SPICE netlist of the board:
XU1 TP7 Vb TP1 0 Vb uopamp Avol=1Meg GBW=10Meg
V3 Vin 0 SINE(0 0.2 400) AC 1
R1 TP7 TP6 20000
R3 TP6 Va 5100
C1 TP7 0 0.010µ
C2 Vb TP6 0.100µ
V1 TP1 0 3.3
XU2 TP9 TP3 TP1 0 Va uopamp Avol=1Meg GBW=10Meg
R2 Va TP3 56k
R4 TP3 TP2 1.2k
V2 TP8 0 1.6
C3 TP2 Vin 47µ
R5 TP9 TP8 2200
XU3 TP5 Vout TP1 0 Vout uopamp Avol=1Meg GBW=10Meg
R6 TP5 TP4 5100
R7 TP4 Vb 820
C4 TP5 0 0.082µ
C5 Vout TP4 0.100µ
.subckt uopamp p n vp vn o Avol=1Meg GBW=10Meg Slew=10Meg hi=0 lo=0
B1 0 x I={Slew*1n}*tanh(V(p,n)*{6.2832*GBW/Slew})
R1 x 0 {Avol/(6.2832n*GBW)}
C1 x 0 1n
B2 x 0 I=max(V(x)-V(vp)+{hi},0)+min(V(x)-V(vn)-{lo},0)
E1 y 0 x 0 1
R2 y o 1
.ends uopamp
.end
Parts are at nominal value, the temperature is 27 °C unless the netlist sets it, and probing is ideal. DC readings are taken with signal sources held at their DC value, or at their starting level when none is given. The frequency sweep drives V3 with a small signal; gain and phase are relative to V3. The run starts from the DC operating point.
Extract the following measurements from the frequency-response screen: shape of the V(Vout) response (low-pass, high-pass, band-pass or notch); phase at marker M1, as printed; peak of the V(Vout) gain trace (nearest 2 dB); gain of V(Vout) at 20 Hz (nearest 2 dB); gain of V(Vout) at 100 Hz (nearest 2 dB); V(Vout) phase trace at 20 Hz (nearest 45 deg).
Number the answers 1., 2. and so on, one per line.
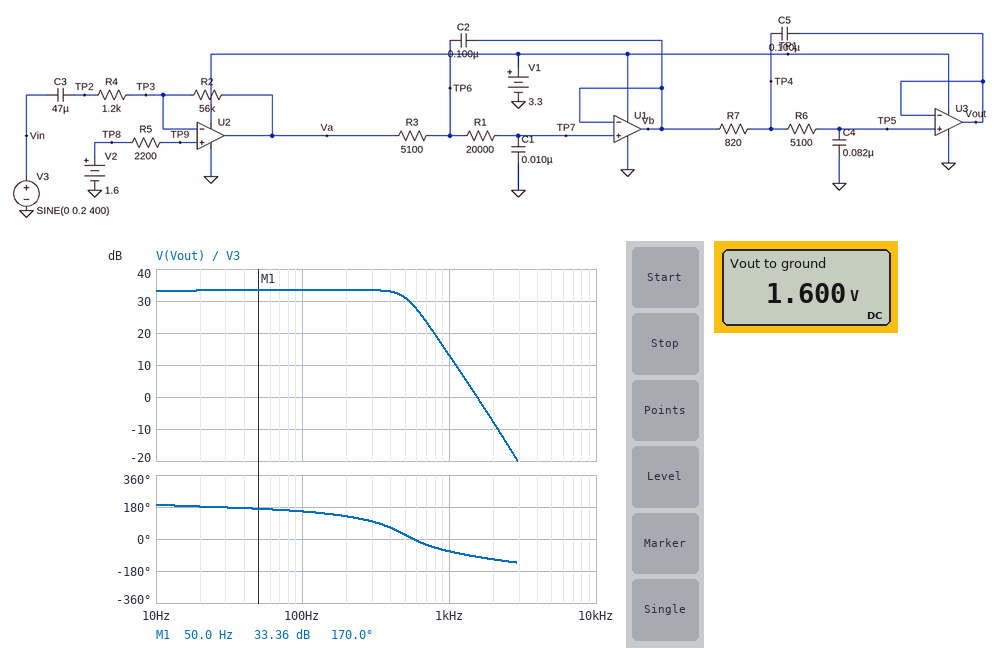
1. low-pass
2. 170.0 deg
3. 34 dB
4. 34 dB
5. 34 dB
6. 180 deg
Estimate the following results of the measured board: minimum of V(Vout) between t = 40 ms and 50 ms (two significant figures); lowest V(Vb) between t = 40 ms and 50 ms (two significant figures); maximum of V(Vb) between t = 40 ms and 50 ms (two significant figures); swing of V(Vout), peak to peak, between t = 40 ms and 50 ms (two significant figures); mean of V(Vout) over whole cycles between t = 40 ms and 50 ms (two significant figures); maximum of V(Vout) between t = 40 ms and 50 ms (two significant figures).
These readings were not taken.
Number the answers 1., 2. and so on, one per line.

1. 300 mV
2. -9.9 mV
3. 3.3 V
4. 2.7 V
5. 1.6 V
6. 3.0 V
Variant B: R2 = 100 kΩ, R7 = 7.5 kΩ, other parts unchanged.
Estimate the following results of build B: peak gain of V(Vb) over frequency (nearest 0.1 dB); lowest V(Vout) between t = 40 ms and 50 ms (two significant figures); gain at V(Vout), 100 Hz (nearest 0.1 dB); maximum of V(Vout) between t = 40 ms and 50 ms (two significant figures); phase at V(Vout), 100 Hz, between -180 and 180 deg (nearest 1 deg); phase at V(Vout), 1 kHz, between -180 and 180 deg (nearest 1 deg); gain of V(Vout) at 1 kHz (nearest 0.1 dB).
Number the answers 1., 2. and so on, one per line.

1. 41.2 dB
2. 920 mV
3. 37.9 dB
4. 2.4 V
5. 136 deg
6. -123 deg
7. 5.4 dB
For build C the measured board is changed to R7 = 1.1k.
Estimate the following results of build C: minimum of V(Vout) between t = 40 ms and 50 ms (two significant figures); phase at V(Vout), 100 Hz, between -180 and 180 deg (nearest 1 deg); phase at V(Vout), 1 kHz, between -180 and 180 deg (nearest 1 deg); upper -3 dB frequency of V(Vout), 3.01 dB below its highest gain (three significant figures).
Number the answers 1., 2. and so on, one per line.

1. 310 mV
2. 154 deg
3. -77 deg
4. 517 Hz
